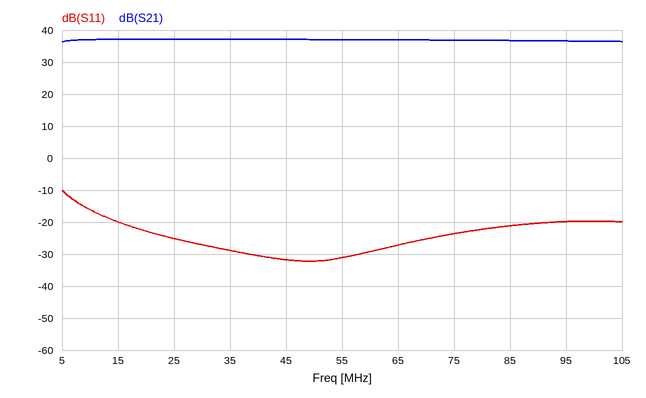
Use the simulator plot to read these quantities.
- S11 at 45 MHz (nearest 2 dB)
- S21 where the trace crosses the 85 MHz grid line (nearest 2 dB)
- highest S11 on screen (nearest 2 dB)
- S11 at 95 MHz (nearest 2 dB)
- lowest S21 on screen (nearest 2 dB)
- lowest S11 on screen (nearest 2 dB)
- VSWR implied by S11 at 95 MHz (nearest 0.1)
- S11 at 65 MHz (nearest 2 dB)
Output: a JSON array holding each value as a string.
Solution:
["-32 dB", "36 dB", "-10 dB", "-20 dB", "36 dB", "-32 dB", "1.2", "-28 dB"]
